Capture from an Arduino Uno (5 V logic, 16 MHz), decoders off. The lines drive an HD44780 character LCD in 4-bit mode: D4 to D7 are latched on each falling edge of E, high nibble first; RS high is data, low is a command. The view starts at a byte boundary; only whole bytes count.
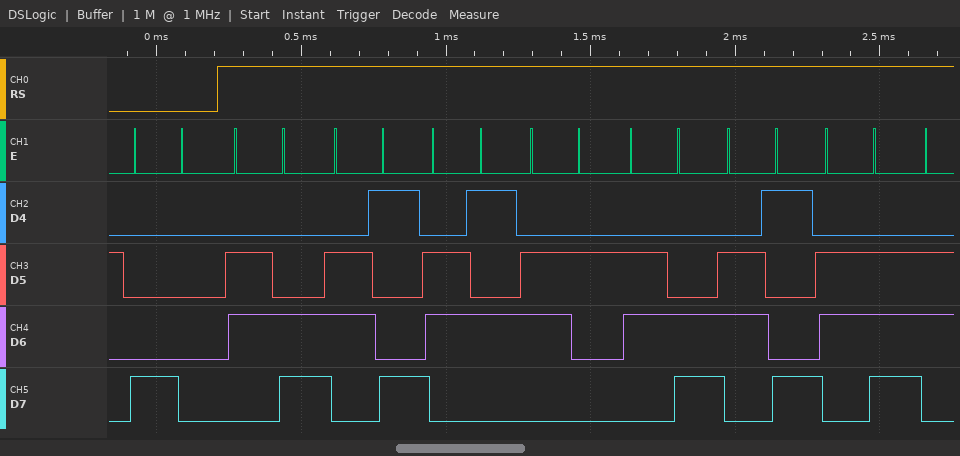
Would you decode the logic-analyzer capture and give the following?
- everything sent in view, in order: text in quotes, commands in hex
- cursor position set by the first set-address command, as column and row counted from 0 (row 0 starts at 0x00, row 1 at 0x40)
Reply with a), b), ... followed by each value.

a) 0x80 "lieblin"
b) column 0, row 0
